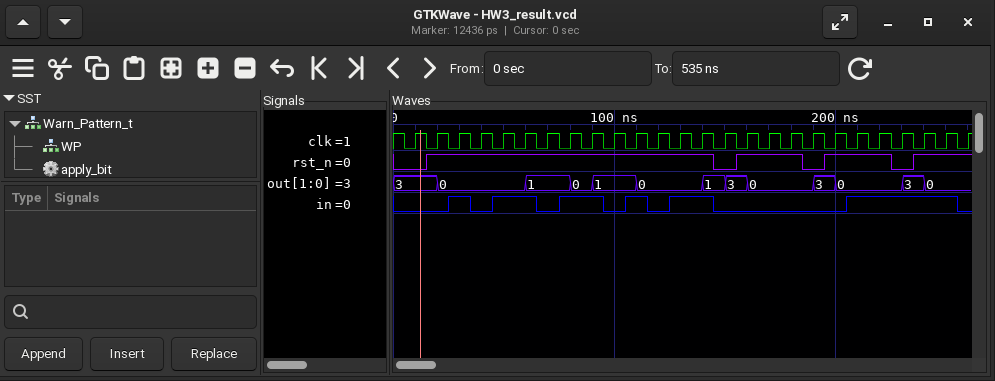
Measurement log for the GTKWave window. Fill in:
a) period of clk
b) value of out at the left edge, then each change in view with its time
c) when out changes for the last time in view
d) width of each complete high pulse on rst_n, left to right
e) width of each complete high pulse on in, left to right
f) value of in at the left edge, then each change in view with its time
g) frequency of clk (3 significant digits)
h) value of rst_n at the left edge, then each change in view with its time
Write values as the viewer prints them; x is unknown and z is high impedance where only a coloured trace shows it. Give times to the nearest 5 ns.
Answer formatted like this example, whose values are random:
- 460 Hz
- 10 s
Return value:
- 10 ns
- 3, 0 at 20 ns, 1 at 60 ns, 0 at 80 ns, 1 at 90 ns, 0 at 110 ns, 1 at 140 ns, 3 at 150 ns, 0 at 160 ns, 3 at 190 ns, 0 at 200 ns, 3 at 230 ns, 0 at 240 ns
- 240 ns
- 130 ns, 30 ns, 30 ns
- 10 ns, 20 ns, 20 ns, 10 ns, 20 ns, 50 ns
- 0, 1 at 25 ns, 0 at 35 ns, 1 at 45 ns, 0 at 65 ns, 1 at 75 ns, 0 at 95 ns, 1 at 105 ns, 0 at 115 ns, 1 at 125 ns, 0 at 145 ns, 1 at 205 ns, 0 at 255 ns
- 100 MHz
- 0, 1 at 15 ns, 0 at 145 ns, 1 at 155 ns, 0 at 185 ns, 1 at 195 ns, 0 at 225 ns, 1 at 235 ns
